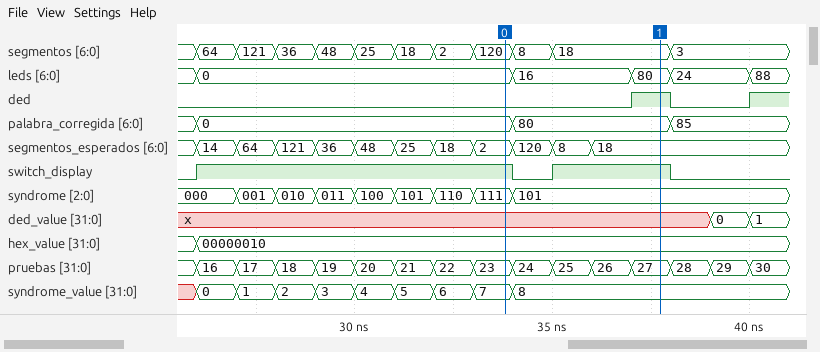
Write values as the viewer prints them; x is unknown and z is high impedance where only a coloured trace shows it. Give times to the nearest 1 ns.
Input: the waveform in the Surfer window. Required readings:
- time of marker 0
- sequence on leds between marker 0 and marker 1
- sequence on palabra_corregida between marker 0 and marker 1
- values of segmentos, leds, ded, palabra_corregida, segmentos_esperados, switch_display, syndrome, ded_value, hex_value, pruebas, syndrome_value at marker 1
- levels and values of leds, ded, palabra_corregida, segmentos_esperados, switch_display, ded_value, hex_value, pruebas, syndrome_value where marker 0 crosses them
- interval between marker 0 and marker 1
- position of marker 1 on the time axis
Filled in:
34 ns
0, 16, 80
0, 80
segmentos=18, leds=80, ded=1, palabra_corregida=80, segmentos_esperados=18, switch_display=1, syndrome=101, ded_value=x, hex_value=00000010, pruebas=27, syndrome_value=8
leds=0, ded=0, palabra_corregida=0, segmentos_esperados=2, switch_display=1, ded_value=x, hex_value=00000010, pruebas=23, syndrome_value=7
4 ns
38 ns
